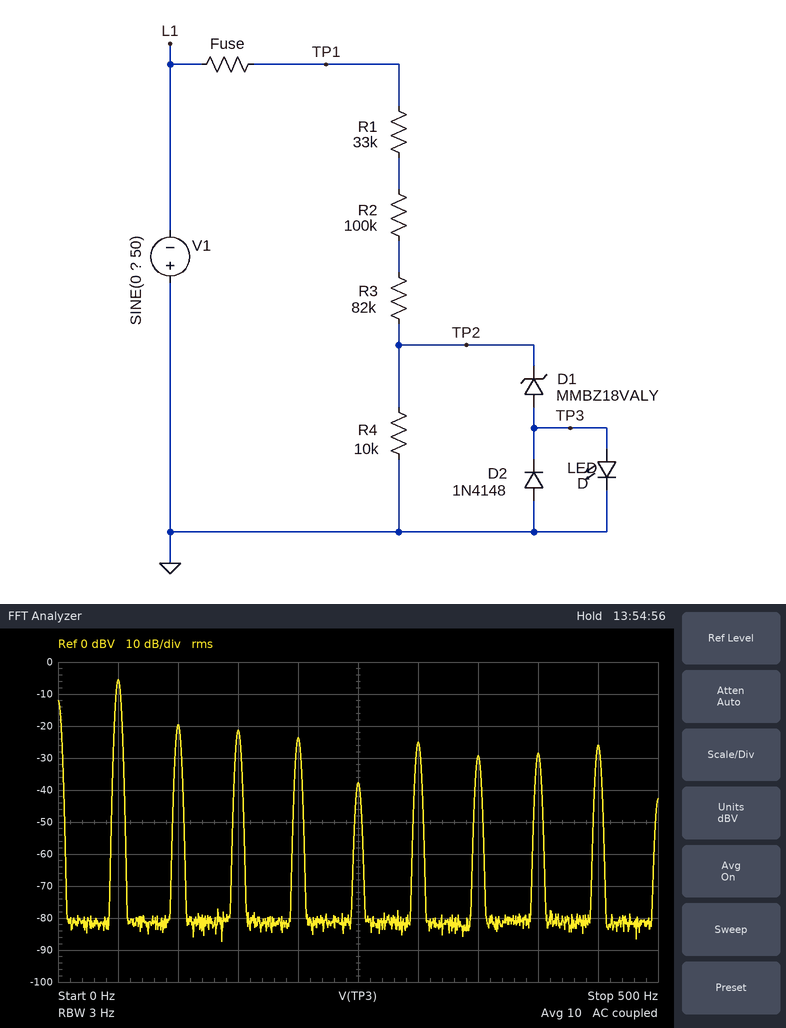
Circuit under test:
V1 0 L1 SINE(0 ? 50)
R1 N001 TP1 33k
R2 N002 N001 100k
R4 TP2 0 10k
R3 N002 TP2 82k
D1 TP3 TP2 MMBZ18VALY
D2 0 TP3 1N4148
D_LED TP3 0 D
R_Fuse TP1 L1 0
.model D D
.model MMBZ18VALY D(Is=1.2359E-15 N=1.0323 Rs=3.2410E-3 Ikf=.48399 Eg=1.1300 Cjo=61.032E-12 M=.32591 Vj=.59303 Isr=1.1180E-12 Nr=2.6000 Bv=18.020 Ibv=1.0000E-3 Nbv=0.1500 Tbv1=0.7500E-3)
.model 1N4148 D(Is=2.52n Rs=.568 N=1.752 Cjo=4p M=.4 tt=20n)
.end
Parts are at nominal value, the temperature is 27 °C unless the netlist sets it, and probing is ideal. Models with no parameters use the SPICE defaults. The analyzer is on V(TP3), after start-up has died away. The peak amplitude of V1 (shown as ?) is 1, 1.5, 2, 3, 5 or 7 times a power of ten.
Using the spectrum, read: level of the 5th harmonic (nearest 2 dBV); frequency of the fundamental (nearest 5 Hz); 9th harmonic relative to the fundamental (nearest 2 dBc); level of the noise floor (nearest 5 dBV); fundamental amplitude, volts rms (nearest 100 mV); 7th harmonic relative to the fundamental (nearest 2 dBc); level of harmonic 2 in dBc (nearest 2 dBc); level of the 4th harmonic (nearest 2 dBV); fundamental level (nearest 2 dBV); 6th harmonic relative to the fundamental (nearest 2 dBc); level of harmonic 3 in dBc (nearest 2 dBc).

-38 dBV
50 Hz
-20 dBc
-80 dBV
500 mV
-24 dBc
-14 dBc
-24 dBV
-6 dBV
-20 dBc
-16 dBc
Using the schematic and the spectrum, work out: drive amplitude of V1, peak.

700 V
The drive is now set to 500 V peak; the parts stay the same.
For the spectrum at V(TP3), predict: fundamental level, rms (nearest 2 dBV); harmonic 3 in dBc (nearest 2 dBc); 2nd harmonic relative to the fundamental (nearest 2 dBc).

-6 dBV
-24 dBc
-12 dBc
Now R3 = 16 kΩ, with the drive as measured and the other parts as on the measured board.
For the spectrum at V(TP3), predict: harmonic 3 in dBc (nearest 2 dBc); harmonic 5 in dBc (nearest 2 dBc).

-12 dBc
-22 dBc
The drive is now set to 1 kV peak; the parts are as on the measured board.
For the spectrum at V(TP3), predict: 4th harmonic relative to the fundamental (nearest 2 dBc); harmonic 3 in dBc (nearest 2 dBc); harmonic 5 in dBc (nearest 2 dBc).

-20 dBc
-12 dBc
-22 dBc
